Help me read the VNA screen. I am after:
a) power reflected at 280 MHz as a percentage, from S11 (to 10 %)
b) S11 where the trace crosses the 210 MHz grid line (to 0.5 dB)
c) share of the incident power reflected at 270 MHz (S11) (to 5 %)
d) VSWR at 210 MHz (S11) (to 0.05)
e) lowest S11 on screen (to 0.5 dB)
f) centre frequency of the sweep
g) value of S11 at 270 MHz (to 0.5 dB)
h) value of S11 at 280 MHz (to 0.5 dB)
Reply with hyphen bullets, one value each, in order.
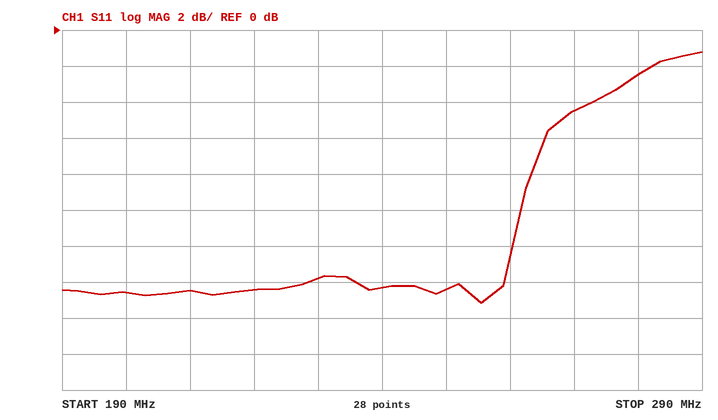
- 60 %
- -14.5 dB
- 35 %
- 1.45
- -15.0 dB
- 240 MHz
- -4.5 dB
- -2.5 dB
